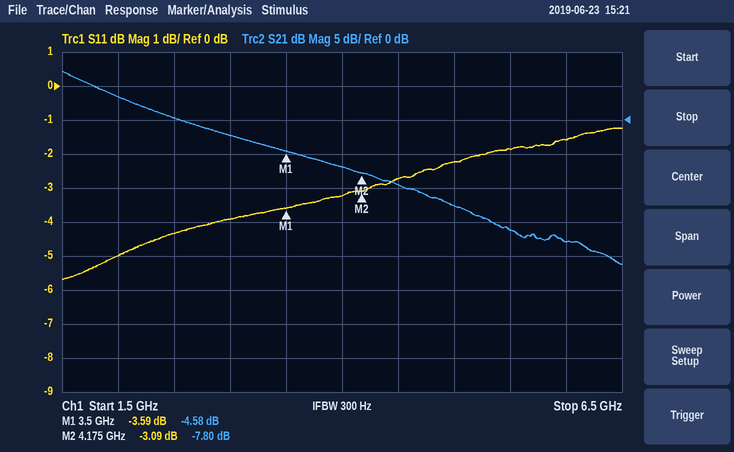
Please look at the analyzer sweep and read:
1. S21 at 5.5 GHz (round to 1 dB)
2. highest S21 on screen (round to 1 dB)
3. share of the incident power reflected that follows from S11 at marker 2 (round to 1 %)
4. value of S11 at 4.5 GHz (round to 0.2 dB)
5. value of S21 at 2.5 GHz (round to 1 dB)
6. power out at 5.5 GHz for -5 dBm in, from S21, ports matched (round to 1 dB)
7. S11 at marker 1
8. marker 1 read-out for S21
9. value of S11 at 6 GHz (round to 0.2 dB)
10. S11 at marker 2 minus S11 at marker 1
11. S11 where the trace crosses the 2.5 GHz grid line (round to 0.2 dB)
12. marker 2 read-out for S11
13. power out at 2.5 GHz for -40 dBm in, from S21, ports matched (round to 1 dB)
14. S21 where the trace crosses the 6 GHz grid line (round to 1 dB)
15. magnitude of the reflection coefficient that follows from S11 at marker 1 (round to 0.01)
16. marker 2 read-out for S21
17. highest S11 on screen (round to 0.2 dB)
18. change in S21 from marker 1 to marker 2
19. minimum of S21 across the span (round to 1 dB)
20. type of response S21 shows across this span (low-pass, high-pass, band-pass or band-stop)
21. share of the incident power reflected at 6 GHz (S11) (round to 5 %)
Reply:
-16 dB
7 dB
49 %
-2.8 dB
0 dB
-21 dBm
-3.59 dB
-4.58 dB
-1.6 dB
0.50 dB
-4.4 dB
-3.09 dB
-40 dBm
-18 dB
0.66
-7.80 dB
-1.2 dB
-3.22 dB
-21 dB
low-pass
70 %
